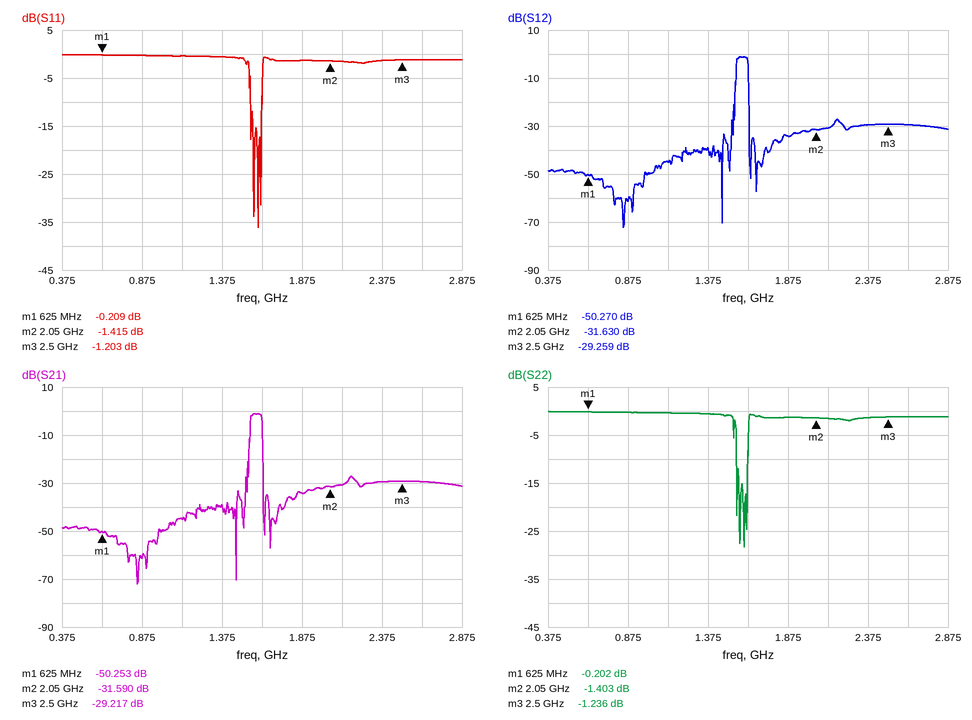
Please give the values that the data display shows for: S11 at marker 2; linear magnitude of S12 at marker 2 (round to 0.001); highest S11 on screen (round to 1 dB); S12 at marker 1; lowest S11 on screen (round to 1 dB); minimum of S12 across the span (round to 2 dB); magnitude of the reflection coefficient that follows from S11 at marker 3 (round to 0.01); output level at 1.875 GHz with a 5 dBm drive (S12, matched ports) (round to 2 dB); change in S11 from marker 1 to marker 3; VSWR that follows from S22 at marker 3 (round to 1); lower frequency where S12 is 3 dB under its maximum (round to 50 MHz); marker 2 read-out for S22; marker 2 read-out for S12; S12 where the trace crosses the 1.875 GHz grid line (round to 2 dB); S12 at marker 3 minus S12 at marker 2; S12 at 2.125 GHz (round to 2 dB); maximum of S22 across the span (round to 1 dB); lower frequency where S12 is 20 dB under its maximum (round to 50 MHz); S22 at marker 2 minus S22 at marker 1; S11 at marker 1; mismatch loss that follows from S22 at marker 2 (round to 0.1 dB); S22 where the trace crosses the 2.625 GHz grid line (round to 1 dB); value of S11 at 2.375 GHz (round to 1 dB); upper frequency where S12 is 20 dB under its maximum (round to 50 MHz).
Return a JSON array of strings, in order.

["-1.415 dB", "0.026", "0 dB", "-50.270 dB", "-36 dB", "-72 dB", "0.87", "-30 dBm", "-0.994 dB", "14", "1.55 GHz", "-1.403 dB", "-31.630 dB", "-34 dB", "2.371 dB", "-30 dB", "0 dB", "1.55 GHz", "-1.201 dB", "-0.209 dB", "5.6 dB", "-1 dB", "-1 dB", "1.65 GHz"]
